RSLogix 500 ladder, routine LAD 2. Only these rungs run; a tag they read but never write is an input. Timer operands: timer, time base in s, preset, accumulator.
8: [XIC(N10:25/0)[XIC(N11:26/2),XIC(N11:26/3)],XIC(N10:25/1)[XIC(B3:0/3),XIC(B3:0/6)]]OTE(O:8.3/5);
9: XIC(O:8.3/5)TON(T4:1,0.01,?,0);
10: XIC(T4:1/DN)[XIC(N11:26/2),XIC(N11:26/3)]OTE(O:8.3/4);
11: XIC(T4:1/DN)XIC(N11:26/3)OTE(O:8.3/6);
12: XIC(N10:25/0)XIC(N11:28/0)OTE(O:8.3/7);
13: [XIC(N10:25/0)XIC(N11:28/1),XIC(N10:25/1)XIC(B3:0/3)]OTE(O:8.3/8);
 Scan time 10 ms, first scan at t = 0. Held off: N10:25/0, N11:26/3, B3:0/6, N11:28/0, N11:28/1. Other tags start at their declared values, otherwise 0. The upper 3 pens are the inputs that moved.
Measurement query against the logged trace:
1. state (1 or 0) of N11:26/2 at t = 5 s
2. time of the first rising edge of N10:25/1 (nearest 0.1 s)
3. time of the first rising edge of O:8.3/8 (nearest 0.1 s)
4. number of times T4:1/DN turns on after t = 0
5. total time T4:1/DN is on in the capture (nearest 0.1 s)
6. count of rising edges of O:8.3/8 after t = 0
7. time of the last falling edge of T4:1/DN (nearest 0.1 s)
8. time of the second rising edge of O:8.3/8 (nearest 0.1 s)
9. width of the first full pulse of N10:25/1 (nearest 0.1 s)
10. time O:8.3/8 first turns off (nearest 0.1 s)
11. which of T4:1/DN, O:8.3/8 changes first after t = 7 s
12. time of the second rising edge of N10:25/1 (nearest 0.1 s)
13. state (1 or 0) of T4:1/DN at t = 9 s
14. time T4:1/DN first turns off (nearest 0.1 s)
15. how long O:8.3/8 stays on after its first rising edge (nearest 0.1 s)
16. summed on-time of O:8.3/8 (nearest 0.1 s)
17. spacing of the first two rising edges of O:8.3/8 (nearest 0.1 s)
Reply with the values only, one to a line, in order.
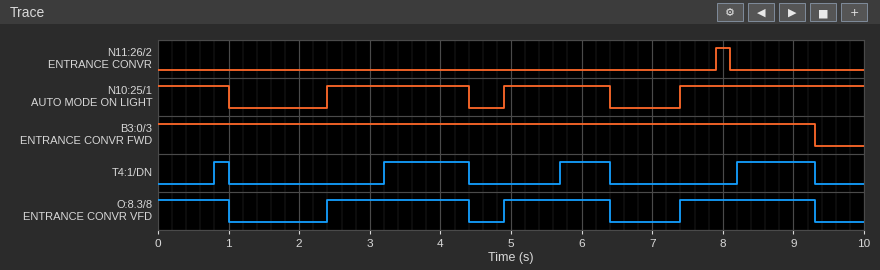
0
2.4 s
2.4 s
4
3.2 s
3
9.3 s
4.9 s
2.0 s
1.0 s
O:8.3/8
4.9 s
1
1.0 s
2.0 s
6.4 s
2.5 s
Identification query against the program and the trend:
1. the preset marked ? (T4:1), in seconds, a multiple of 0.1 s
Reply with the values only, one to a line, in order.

0.8 s
